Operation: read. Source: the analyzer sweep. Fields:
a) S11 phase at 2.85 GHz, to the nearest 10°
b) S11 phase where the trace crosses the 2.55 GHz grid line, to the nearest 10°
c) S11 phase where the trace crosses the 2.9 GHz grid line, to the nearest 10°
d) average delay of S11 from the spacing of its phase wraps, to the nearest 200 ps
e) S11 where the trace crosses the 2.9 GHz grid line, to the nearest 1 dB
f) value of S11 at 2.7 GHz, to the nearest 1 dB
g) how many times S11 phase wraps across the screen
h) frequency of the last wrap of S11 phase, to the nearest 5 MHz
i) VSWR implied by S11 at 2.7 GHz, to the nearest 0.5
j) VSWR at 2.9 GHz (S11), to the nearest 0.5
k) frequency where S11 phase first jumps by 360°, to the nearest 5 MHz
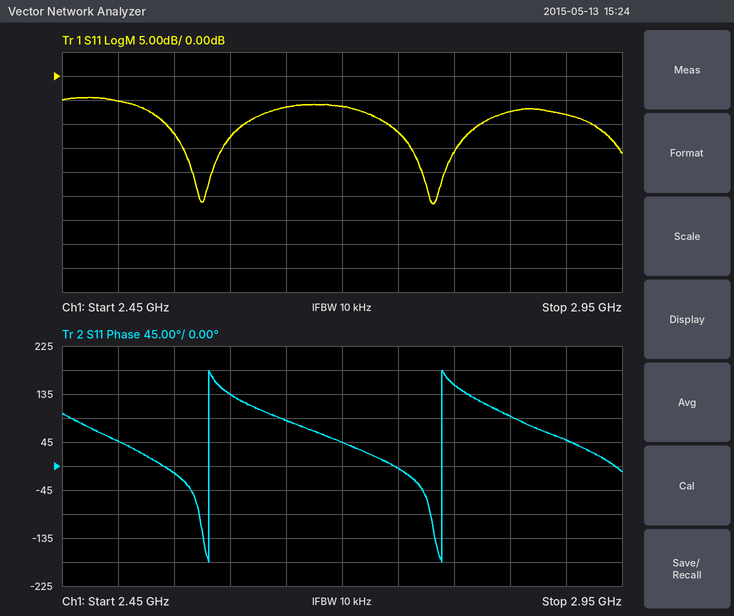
90°
-10°
50°
4.8 ns
-8 dB
-6 dB
2
2.790 GHz
3.0
2.5
2.580 GHz
